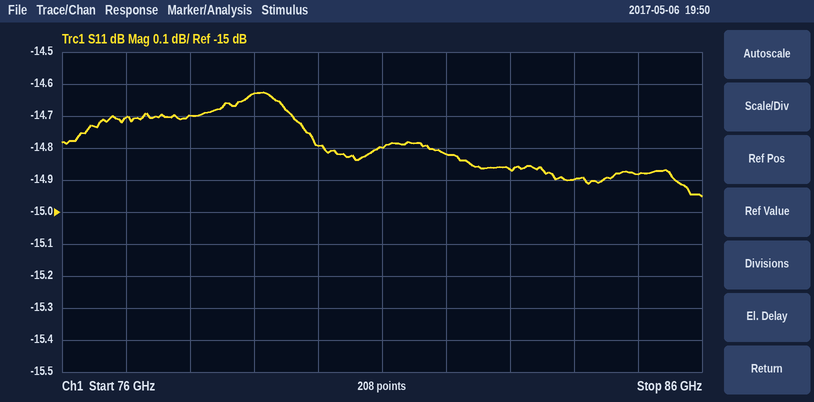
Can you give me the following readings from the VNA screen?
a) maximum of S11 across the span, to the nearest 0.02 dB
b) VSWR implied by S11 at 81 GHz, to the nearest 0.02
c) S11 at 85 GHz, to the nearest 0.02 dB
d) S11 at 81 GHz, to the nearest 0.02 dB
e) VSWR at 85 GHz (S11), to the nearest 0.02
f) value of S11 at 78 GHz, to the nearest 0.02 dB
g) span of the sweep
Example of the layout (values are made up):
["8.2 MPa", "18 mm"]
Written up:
["-14.62 dB", "1.44", "-14.88 dB", "-14.80 dB", "1.44", "-14.70 dB", "10 GHz"]
